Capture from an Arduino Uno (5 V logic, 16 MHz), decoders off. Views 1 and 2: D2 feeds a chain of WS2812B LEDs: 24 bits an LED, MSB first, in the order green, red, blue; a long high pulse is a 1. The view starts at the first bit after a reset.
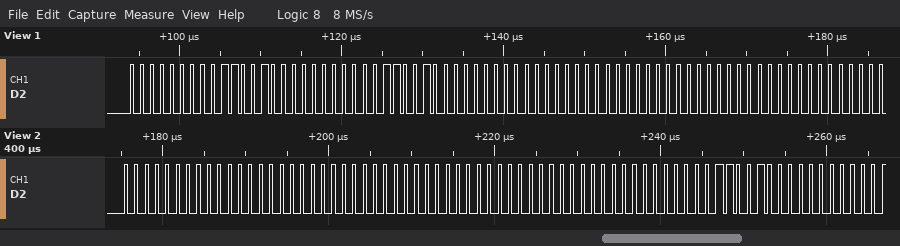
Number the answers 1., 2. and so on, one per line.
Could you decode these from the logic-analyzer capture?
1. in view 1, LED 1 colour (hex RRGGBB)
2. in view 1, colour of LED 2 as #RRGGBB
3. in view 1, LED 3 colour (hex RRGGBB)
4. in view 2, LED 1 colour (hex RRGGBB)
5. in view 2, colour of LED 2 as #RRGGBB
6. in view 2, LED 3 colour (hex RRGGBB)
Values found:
1. #640000
2. #006400
3. #000000
4. #000000
5. #000000
6. #640000
